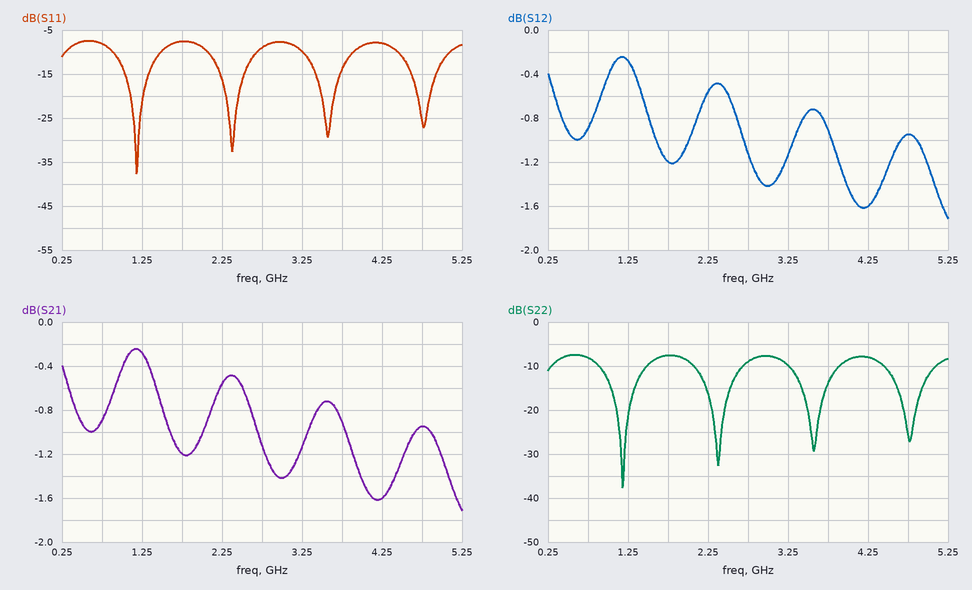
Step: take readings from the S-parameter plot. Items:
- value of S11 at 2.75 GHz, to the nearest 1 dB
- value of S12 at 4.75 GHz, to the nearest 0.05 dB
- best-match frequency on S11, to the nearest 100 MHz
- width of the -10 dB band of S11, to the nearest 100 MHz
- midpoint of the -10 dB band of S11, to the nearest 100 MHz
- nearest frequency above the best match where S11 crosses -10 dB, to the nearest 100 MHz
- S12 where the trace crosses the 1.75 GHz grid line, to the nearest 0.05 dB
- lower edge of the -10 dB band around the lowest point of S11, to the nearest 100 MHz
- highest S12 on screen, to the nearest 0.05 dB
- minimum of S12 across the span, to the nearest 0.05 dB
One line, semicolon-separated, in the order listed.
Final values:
-9 dB; -0.95 dB; 1.2 GHz; 600 MHz; 1.2 GHz; 1.5 GHz; -1.20 dB; 900 MHz; -0.25 dB; -1.70 dB
